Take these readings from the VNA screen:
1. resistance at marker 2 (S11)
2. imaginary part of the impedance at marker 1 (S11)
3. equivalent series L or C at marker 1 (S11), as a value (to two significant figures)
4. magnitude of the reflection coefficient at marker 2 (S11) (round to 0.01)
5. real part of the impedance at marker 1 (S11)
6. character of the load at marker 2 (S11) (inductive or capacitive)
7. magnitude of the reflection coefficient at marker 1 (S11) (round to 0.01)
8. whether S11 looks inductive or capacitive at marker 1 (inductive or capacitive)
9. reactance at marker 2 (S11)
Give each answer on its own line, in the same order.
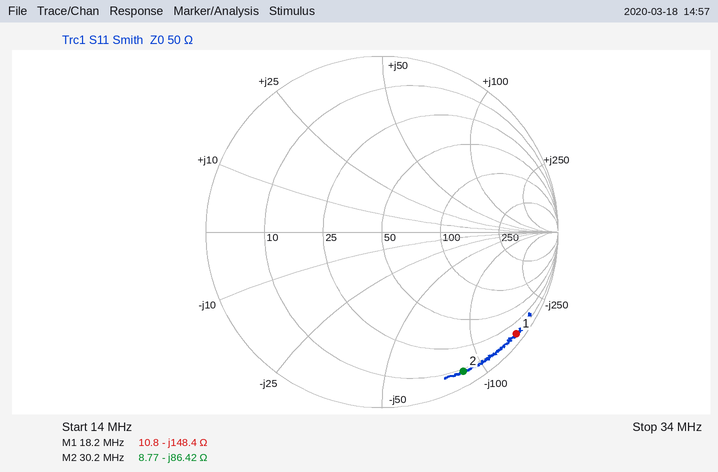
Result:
8.77 Ω
-148.4 Ω
59 pF
0.92
10.8 Ω
capacitive
0.96
capacitive
-86.42 Ω
